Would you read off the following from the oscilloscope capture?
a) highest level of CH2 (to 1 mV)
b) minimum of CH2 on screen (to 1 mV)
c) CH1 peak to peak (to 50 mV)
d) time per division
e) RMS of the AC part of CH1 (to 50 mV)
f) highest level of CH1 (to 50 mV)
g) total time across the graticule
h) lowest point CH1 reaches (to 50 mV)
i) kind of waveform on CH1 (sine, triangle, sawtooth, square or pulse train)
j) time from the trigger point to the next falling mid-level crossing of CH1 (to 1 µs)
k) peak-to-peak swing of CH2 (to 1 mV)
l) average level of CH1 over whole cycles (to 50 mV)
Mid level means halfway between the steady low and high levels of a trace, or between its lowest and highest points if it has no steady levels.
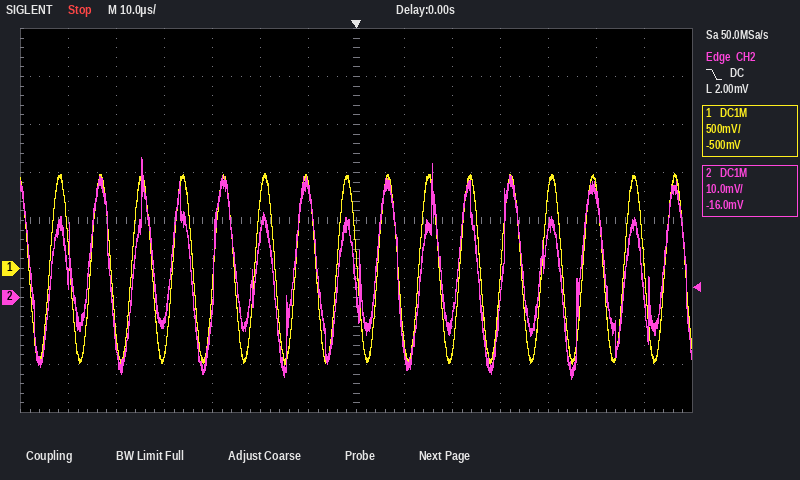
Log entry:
29 mV
-17 mV
2.00 V
10 µs
700 mV
1.00 V
140 µs
-1.00 V
sine
9 µs
46 mV
0 mV
